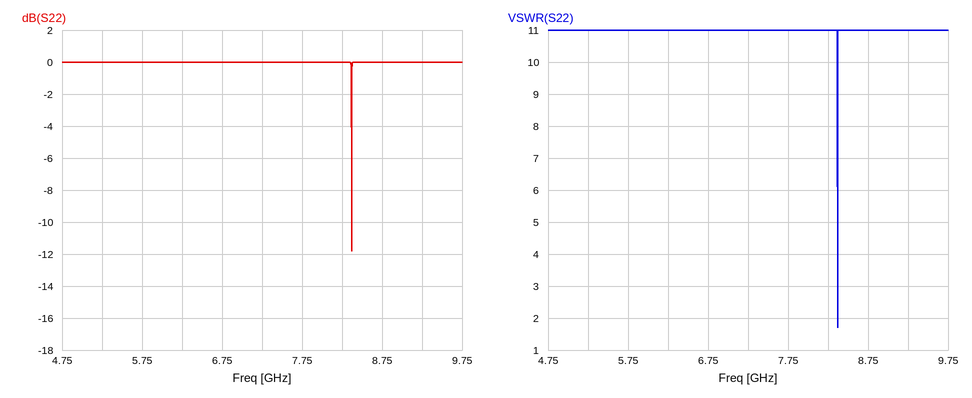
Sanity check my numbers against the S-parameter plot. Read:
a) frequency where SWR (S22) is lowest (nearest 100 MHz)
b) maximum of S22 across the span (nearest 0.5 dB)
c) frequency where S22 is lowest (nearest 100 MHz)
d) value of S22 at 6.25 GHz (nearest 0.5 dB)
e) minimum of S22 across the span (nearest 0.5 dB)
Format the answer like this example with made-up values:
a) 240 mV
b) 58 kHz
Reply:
a) 8.4 GHz
b) 0.0 dB
c) 8.4 GHz
d) 0.0 dB
e) -12.0 dB
